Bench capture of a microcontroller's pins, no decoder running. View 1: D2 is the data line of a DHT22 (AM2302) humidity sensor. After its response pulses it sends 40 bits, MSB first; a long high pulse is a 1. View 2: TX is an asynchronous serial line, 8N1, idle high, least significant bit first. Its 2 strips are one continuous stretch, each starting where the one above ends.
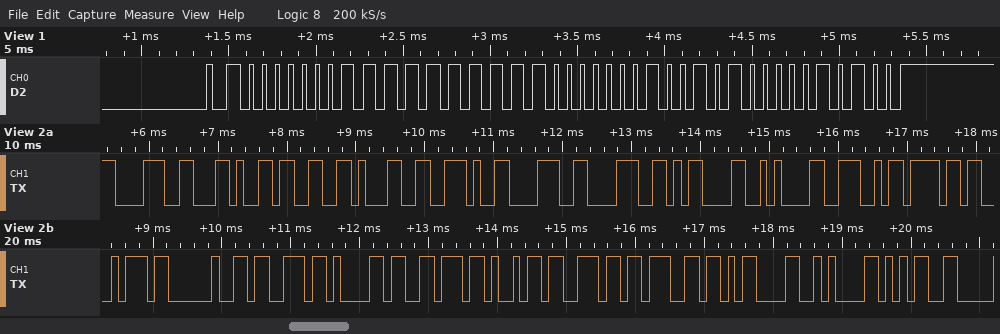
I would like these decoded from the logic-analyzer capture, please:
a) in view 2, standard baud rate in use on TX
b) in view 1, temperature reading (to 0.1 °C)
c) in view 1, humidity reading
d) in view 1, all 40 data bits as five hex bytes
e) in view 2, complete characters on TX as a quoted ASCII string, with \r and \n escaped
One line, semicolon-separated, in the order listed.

9600 baud; -14.8 °C; 51.1 %; 01 FF 80 94 14; "8,31.88\r\nNot saving\r\n5"
